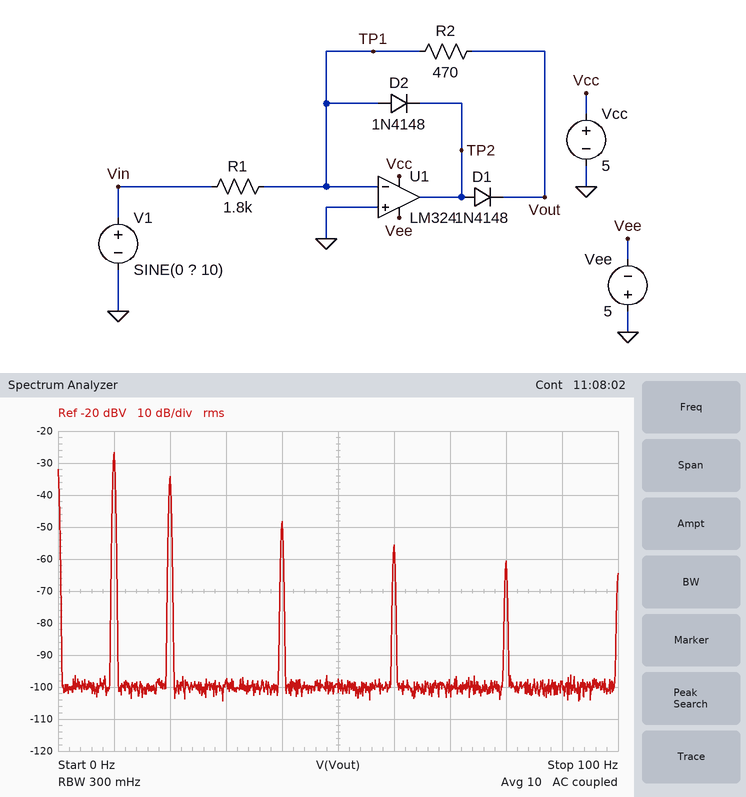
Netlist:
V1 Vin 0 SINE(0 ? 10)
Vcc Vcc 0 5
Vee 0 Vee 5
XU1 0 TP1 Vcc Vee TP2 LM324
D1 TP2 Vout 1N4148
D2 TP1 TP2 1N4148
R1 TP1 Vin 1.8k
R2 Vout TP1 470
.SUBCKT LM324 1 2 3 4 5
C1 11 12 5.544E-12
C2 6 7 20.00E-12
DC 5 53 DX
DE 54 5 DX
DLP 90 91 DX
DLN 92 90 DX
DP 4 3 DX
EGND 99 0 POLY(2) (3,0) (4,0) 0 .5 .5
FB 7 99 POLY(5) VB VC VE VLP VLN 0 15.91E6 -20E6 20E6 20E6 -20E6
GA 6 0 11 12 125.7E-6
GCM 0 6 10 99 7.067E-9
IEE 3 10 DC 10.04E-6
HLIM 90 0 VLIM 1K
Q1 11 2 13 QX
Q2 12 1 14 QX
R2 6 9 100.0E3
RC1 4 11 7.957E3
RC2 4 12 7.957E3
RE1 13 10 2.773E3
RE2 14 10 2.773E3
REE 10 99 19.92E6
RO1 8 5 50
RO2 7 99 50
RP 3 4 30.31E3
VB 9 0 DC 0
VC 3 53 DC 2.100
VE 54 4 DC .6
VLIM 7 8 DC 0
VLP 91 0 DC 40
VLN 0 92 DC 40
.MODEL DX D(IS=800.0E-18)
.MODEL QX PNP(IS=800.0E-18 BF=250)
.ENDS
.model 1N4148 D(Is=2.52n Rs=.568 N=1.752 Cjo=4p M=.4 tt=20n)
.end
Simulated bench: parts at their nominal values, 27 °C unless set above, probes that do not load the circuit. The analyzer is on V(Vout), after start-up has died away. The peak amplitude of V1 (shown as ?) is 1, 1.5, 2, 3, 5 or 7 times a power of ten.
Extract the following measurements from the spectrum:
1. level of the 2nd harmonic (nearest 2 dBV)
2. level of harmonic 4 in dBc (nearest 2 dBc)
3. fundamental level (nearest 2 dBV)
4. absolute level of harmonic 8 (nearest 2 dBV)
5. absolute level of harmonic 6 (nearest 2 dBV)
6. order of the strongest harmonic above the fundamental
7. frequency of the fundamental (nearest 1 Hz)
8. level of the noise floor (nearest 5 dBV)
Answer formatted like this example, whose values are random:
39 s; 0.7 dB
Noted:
-34 dBV; -22 dBc; -26 dBV; -60 dBV; -56 dBV; 2; 10 Hz; -100 dBV
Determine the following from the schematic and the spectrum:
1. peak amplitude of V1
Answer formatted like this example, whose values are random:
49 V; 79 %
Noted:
500 mV
